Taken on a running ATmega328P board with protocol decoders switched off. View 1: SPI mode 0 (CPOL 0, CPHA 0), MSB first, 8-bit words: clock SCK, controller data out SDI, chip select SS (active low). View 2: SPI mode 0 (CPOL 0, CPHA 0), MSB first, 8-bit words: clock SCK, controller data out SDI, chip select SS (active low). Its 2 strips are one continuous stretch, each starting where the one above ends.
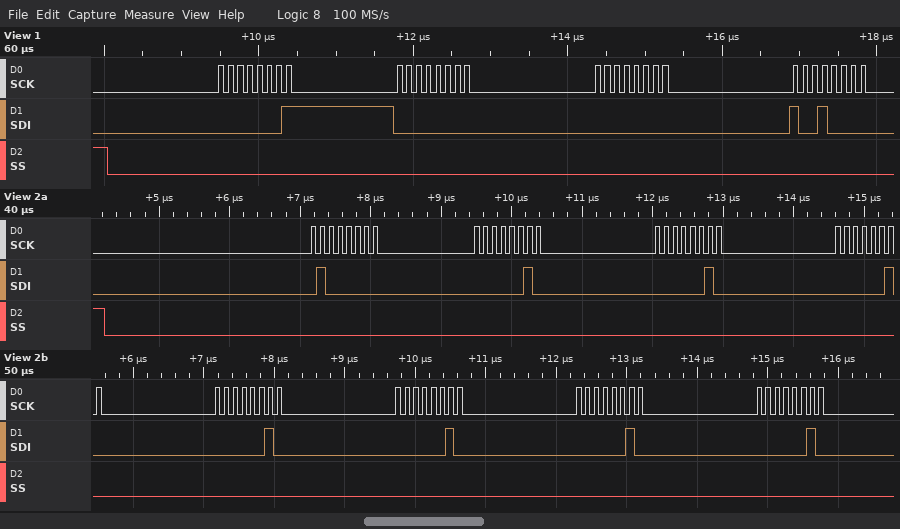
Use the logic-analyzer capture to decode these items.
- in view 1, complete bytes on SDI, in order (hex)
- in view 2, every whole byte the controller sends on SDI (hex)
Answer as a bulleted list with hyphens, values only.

- 0x01 0x00 0x00 0x90
- 40 02 02 02 02 02 02 02
